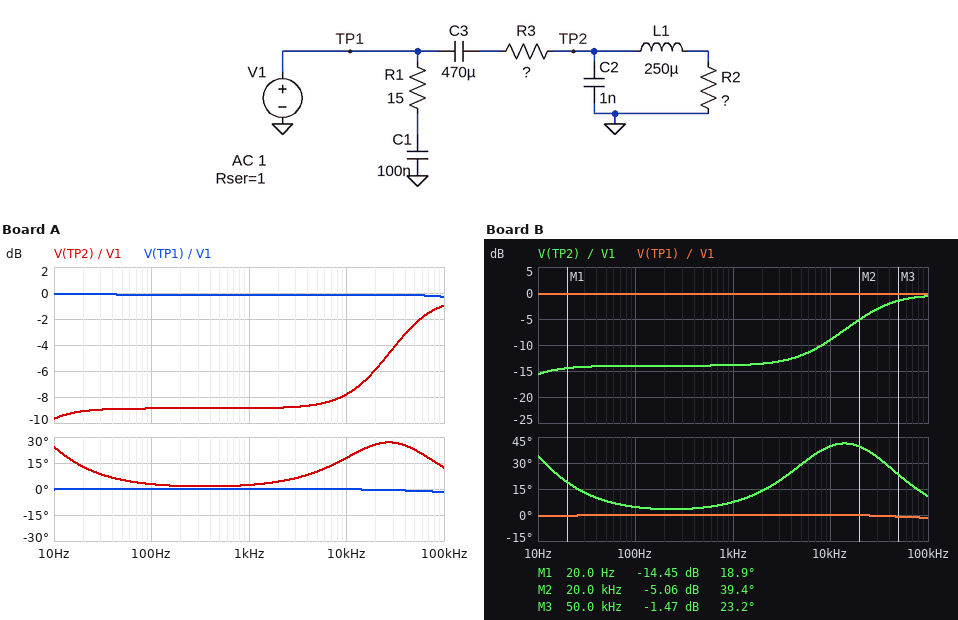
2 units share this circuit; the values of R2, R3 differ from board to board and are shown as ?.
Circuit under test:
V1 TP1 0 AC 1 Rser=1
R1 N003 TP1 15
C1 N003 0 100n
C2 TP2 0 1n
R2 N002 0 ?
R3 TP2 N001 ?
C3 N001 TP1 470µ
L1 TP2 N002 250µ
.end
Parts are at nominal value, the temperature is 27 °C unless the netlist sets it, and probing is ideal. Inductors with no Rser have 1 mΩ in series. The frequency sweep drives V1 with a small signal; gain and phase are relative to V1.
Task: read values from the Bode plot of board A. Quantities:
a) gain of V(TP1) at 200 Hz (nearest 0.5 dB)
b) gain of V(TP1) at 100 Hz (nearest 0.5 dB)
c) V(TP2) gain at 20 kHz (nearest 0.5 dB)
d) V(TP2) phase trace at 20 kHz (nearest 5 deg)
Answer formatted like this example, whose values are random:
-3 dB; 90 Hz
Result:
0 dB; 0 dB; -6.0 dB; 25 deg
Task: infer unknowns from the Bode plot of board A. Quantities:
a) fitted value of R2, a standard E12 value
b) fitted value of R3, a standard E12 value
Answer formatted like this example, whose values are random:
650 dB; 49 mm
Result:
27 Ω; 47 Ω
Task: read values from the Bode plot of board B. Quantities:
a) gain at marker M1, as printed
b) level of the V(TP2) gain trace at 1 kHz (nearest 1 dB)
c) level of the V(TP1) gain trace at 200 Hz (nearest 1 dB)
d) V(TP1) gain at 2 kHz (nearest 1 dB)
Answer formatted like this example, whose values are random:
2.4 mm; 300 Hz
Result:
-14.45 dB; -14 dB; 0 dB; 0 dB
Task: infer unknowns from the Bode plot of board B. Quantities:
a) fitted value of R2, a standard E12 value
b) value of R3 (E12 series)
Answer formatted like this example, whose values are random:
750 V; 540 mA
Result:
10 Ω; 39 Ω
